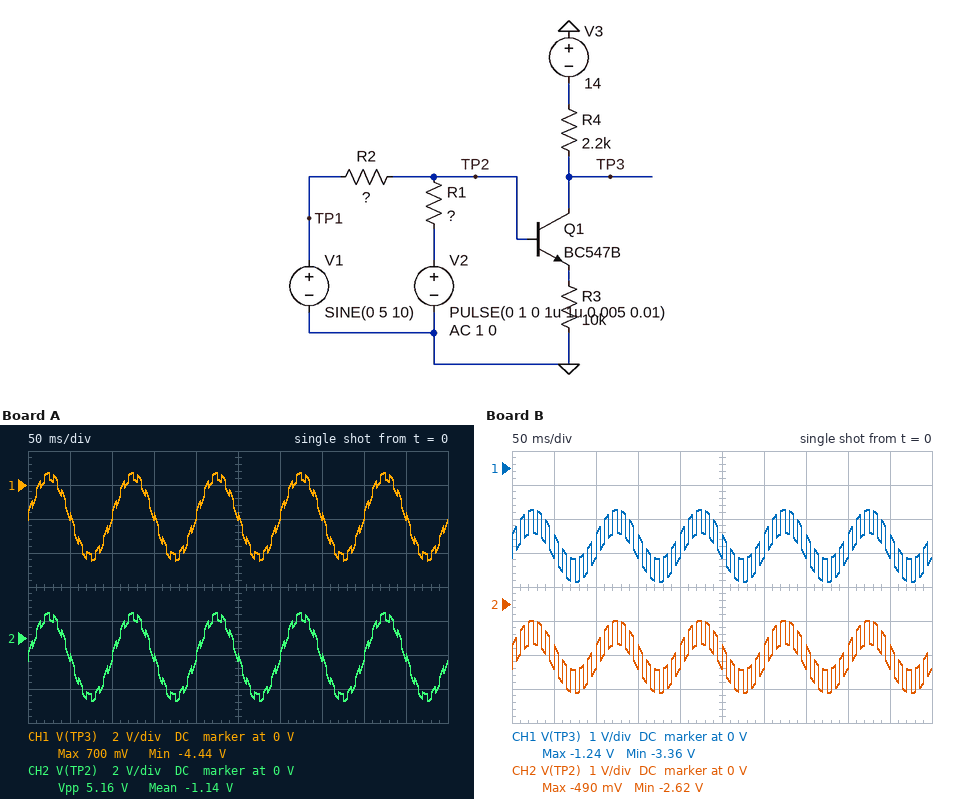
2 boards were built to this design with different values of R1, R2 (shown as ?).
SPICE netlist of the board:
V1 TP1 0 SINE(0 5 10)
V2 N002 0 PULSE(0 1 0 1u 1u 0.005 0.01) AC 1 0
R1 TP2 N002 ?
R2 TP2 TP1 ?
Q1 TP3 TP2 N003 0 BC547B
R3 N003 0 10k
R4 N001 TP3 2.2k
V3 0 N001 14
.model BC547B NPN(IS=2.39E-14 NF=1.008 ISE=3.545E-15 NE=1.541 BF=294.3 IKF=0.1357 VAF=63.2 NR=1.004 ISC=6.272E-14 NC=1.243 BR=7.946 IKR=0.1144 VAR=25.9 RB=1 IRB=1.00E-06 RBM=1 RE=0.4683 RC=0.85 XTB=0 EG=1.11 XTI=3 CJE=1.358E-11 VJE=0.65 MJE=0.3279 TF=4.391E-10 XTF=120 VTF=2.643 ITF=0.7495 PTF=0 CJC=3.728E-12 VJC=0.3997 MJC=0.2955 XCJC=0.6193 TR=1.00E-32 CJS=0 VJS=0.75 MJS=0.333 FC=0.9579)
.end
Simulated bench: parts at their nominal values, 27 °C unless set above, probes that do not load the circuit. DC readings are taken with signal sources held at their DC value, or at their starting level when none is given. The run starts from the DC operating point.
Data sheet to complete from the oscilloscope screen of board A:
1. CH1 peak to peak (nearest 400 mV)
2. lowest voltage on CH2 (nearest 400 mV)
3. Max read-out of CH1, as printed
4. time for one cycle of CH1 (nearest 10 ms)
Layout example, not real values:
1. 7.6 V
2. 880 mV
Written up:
1. 5.2 V
2. -3.6 V
3. 700 mV
4. 100 ms
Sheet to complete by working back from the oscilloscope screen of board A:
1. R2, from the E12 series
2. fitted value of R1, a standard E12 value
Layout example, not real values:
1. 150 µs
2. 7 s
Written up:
1. 470 Ω
2. 560 Ω
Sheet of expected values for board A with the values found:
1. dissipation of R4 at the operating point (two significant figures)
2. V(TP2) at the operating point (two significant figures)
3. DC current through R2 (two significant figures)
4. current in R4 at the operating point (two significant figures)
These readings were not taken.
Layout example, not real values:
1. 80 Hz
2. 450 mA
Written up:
1. 65 mW
2. -1.3 V
3. 2.8 mA
4. 5.4 mA
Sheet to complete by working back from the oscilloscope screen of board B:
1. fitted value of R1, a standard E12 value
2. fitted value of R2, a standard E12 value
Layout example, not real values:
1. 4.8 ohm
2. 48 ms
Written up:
1. 470 Ω
2. 2.2 kΩ
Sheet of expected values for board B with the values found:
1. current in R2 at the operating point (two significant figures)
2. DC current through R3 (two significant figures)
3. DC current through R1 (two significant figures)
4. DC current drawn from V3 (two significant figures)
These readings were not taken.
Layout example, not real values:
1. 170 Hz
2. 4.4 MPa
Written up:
1. 860 µA
2. 260 µA
3. 4.0 mA
4. 5.2 mA
